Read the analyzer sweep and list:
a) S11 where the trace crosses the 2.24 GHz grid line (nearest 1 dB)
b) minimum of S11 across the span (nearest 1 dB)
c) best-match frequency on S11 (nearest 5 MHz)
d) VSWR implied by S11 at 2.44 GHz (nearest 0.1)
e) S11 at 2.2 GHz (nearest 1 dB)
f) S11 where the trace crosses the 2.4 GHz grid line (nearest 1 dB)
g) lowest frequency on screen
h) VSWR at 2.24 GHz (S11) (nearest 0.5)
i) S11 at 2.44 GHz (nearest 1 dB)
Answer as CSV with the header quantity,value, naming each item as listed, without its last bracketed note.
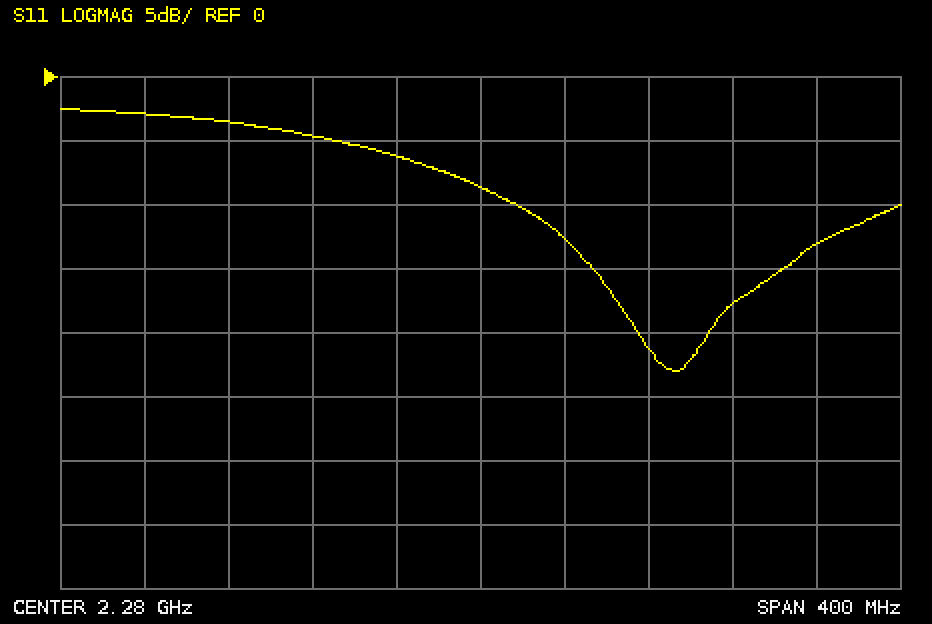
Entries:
quantity,value
S11 where the trace crosses the 2.24 GHz grid line,-6 dB
minimum of S11 across the span,-23 dB
best-match frequency on S11,2.370 GHz
VSWR implied by S11 at 2.44 GHz,1.6
S11 at 2.2 GHz,-5 dB
S11 where the trace crosses the 2.4 GHz grid line,-18 dB
lowest frequency on screen,2.08 GHz
VSWR at 2.24 GHz (S11),3.0
S11 at 2.44 GHz,-13 dB
